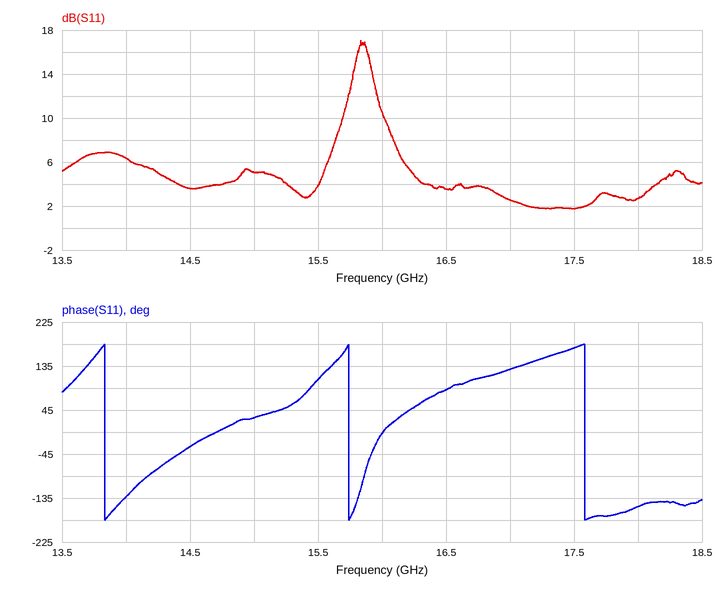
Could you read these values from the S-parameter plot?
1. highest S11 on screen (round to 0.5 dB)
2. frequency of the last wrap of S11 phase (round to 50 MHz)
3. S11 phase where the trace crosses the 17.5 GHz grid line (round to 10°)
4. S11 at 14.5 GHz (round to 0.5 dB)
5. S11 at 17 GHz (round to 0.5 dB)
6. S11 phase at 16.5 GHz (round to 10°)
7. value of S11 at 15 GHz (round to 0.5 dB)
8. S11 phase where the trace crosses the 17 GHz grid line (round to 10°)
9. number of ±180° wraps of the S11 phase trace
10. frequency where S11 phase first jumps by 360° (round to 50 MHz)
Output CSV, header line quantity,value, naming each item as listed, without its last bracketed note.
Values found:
quantity,value
highest S11 on screen,17.0 dB
frequency of the last wrap of S11 phase,17.60 GHz
S11 phase where the trace crosses the 17.5 GHz grid line,170°
S11 at 14.5 GHz,3.5 dB
S11 at 17 GHz,2.5 dB
S11 phase at 16.5 GHz,90°
value of S11 at 15 GHz,5.0 dB
S11 phase where the trace crosses the 17 GHz grid line,130°
number of ±180° wraps of the S11 phase trace,3
frequency where S11 phase first jumps by 360°,13.85 GHz
